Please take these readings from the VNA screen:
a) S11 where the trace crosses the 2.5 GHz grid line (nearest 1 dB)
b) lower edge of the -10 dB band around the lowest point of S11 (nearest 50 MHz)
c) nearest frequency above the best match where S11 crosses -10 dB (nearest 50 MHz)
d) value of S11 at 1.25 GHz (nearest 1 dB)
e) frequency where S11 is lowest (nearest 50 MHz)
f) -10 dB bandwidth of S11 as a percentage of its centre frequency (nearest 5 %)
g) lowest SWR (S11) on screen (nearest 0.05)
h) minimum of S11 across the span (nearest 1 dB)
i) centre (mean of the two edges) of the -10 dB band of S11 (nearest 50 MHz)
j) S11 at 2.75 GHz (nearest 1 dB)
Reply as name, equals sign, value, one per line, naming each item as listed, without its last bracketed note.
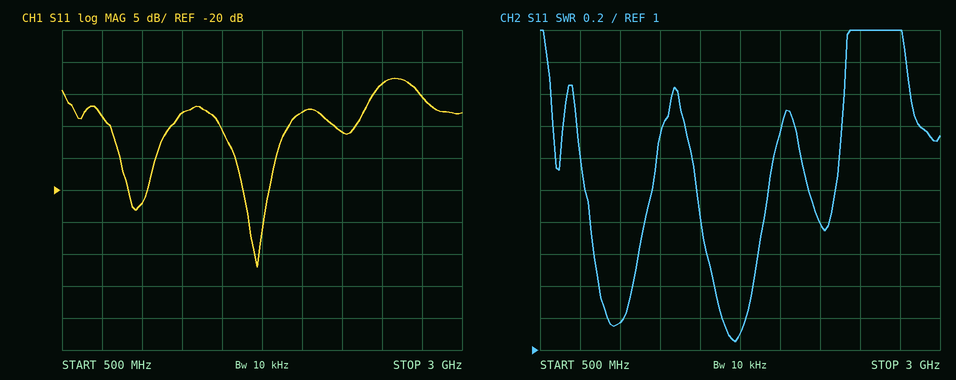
S11 where the trace crosses the 2.5 GHz grid line = -3 dB
lower edge of the -10 dB band around the lowest point of S11 = 1.50 GHz
nearest frequency above the best match where S11 crosses -10 dB = 1.90 GHz
value of S11 at 1.25 GHz = -8 dB
frequency where S11 is lowest = 1.70 GHz
-10 dB bandwidth of S11 as a percentage of its centre frequency = 25 %
lowest SWR (S11) on screen = 1.05
minimum of S11 across the span = -32 dB
centre (mean of the two edges) of the -10 dB band of S11 = 1.70 GHz
S11 at 2.75 GHz = -5 dB
